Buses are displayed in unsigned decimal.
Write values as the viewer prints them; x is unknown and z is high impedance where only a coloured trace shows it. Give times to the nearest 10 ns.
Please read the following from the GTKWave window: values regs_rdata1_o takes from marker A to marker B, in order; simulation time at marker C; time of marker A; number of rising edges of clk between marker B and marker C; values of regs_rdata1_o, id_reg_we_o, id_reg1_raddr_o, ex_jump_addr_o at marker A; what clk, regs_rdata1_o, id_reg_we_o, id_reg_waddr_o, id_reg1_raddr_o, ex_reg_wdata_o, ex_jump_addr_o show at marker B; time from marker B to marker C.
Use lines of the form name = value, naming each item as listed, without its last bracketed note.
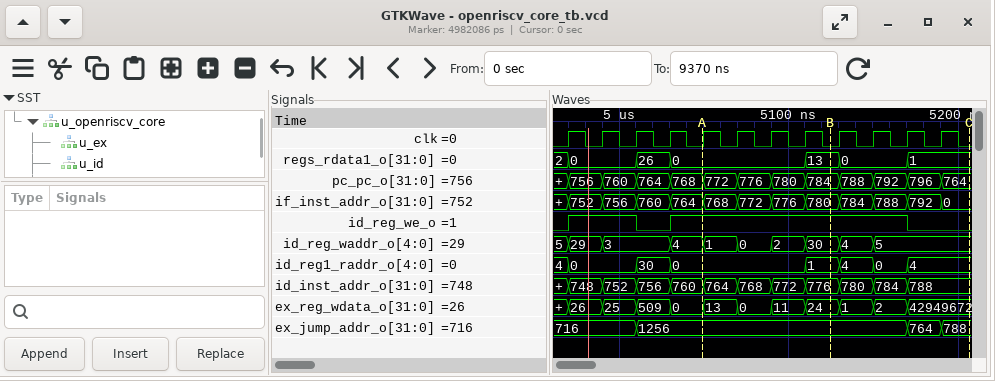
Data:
values regs_rdata1_o takes from marker A to marker B, in order = 0, 13
simulation time at marker C = 5210 ns
time of marker A = 5050 ns
number of rising edges of clk between marker B and marker C = 4
values of regs_rdata1_o, id_reg_we_o, id_reg1_raddr_o, ex_jump_addr_o at marker A = regs_rdata1_o=0, id_reg_we_o=1, id_reg1_raddr_o=0, ex_jump_addr_o=1256
what clk, regs_rdata1_o, id_reg_we_o, id_reg_waddr_o, id_reg1_raddr_o, ex_reg_wdata_o, ex_jump_addr_o show at marker B = clk=0, regs_rdata1_o=13, id_reg_we_o=1, id_reg_waddr_o=30, id_reg1_raddr_o=1, ex_reg_wdata_o=24, ex_jump_addr_o=1256
time from marker B to marker C = 80 ns
